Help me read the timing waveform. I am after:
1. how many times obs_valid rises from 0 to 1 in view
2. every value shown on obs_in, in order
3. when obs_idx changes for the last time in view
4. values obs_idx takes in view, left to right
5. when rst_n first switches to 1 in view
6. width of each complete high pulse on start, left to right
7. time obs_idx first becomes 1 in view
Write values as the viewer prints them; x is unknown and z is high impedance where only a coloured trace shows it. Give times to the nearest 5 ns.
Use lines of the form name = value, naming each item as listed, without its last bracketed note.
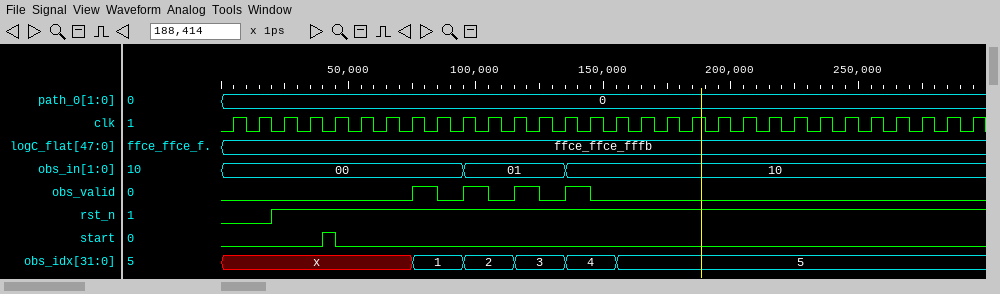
how many times obs_valid rises from 0 to 1 in view = 4
every value shown on obs_in, in order = 00, 01, 10
when obs_idx changes for the last time in view = 155 ns
values obs_idx takes in view, left to right = x, 1, 2, 3, 4, 5
when rst_n first switches to 1 in view = 20 ns
width of each complete high pulse on start, left to right = 5 ns
time obs_idx first becomes 1 in view = 75 ns
